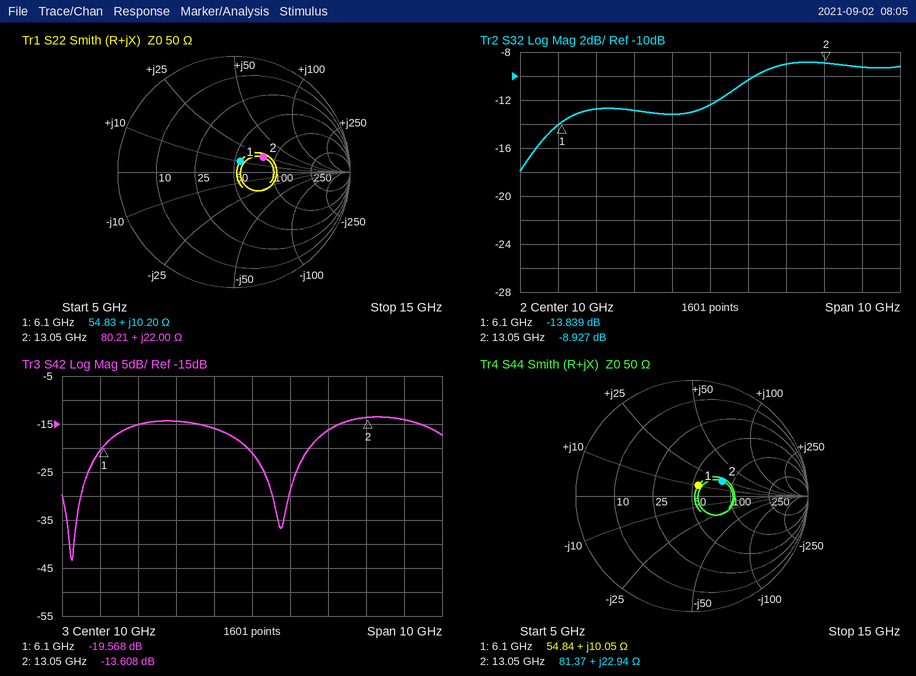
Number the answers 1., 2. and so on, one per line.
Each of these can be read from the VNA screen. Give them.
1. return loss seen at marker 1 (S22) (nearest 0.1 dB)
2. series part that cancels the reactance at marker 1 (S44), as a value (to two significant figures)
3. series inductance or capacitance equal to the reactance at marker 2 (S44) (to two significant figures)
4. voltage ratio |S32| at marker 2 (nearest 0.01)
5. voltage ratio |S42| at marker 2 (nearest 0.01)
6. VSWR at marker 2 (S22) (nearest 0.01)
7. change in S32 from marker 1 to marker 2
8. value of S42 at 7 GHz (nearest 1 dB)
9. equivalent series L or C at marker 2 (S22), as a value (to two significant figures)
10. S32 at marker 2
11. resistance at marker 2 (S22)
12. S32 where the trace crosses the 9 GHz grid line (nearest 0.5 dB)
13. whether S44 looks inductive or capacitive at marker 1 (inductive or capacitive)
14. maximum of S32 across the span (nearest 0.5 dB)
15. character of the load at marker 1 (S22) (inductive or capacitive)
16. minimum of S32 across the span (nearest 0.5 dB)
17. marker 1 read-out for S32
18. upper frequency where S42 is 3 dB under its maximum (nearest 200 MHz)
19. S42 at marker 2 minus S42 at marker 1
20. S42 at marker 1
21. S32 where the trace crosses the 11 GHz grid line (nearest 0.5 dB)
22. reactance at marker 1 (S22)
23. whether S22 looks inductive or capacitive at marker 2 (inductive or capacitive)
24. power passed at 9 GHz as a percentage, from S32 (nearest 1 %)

1. 19.4 dB
2. 2.6 pF
3. 280 pH
4. 0.36
5. 0.21
6. 1.79
7. 4.912 dB
8. -15 dB
9. 270 pH
10. -8.927 dB
11. 80.21 Ω
12. -13.0 dB
13. inductive
14. -9.0 dB
15. inductive
16. -18.0 dB
17. -13.839 dB
18. 14.8 GHz
19. 5.960 dB
20. -19.568 dB
21. -10.5 dB
22. +10.20 Ω
23. inductive
24. 5 %
